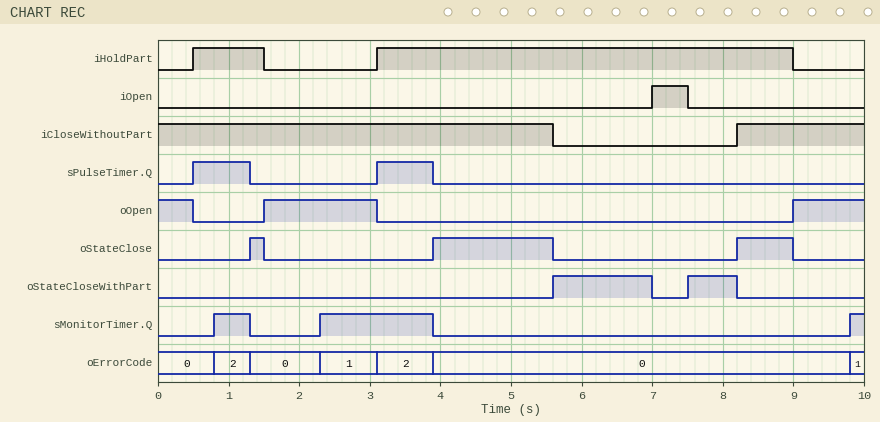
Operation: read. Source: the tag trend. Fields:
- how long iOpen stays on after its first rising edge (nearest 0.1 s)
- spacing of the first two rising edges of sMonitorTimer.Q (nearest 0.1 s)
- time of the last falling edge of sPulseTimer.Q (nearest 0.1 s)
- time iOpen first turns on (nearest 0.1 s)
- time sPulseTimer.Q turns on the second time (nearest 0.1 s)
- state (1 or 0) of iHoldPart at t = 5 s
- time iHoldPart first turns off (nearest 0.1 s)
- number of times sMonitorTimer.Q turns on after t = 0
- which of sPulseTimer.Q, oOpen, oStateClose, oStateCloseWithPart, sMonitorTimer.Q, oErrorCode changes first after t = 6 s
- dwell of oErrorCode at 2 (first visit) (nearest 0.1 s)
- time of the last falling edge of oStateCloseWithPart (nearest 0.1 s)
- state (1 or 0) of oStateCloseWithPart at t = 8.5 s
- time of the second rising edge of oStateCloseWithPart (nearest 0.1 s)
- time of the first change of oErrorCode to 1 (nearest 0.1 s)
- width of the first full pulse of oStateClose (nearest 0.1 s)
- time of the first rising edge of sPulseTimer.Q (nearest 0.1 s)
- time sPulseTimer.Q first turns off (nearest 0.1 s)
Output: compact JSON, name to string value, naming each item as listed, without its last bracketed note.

{"how long iOpen stays on after its first rising edge": "0.5 s", "spacing of the first two rising edges of sMonitorTimer.Q": "1.5 s", "time of the last falling edge of sPulseTimer.Q": "3.9 s", "time iOpen first turns on": "7.0 s", "time sPulseTimer.Q turns on the second time": "3.1 s", "state (1 or 0) of iHoldPart at t = 5 s": "1", "time iHoldPart first turns off": "1.5 s", "number of times sMonitorTimer.Q turns on after t = 0": "3", "which of sPulseTimer.Q, oOpen, oStateClose, oStateCloseWithPart, sMonitorTimer.Q, oErrorCode changes first after t = 6 s": "oStateCloseWithPart", "dwell of oErrorCode at 2 (first visit)": "0.5 s", "time of the last falling edge of oStateCloseWithPart": "8.2 s", "state (1 or 0) of oStateCloseWithPart at t = 8.5 s": "0", "time of the second rising edge of oStateCloseWithPart": "7.5 s", "time of the first change of oErrorCode to 1": "2.3 s", "width of the first full pulse of oStateClose": "0.2 s", "time of the first rising edge of sPulseTimer.Q": "0.5 s", "time sPulseTimer.Q first turns off": "1.3 s"}
